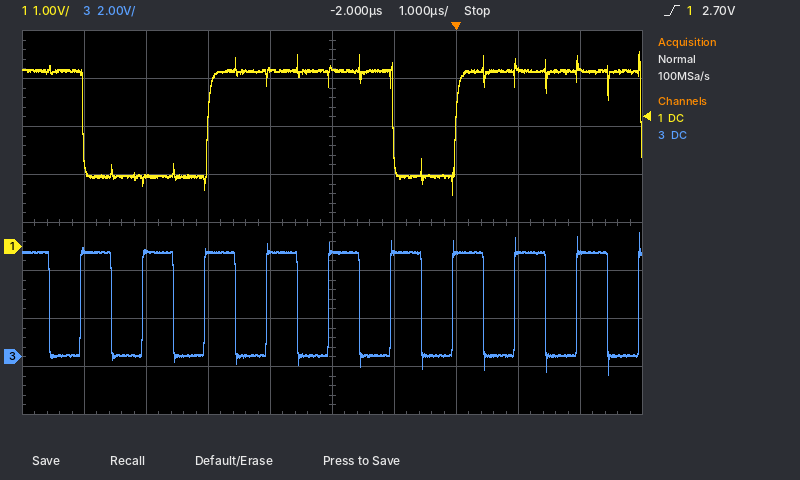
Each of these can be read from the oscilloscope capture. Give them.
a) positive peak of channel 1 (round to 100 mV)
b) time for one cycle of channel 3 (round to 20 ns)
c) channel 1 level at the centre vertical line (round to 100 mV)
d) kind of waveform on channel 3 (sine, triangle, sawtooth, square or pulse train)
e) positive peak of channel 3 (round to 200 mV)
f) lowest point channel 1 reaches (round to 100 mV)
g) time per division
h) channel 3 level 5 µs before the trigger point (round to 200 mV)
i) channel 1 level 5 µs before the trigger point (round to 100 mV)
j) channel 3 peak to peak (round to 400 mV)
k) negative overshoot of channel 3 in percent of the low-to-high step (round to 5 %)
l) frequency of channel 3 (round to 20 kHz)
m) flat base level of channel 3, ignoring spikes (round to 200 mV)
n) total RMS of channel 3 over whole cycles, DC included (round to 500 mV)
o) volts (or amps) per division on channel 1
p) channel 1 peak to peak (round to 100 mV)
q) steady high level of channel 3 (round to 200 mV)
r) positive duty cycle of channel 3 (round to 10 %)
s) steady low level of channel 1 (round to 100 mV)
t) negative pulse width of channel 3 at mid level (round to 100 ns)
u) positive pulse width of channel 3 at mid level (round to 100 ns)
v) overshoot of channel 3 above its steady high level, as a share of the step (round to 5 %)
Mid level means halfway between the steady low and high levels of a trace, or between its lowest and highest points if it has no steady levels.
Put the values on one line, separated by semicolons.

4.1 V; 1.00 µs; 3.7 V; square; 5.2 V; 1.1 V; 1 µs; 4.4 V; 1.4 V; 6.0 V; 20 %; 1.00 MHz; 0.0 V; 3.0 V; 1 V; 3.0 V; 4.4 V; 50 %; 1.5 V; 500 ns; 500 ns; 20 %
